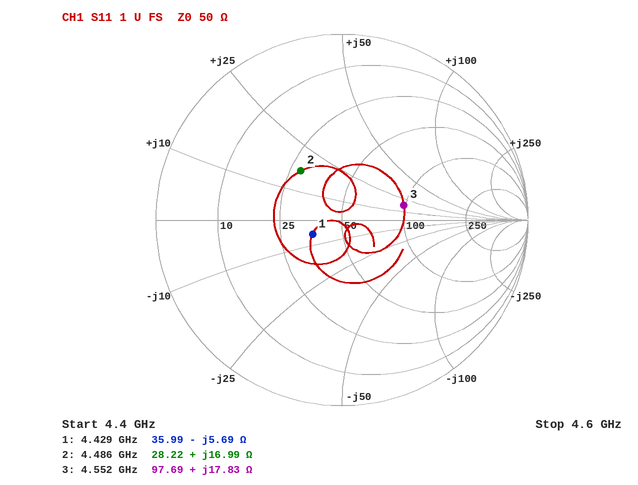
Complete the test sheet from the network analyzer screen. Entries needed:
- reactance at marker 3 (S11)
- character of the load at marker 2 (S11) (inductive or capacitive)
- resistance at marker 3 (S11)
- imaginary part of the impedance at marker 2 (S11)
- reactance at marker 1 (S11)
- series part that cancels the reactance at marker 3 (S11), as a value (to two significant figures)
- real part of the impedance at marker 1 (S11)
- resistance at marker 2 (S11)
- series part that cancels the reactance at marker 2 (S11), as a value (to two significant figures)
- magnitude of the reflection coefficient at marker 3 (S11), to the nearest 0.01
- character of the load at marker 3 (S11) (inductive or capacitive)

+17.83 Ω
inductive
97.69 Ω
+16.99 Ω
-5.69 Ω
2.0 pF
35.99 Ω
28.22 Ω
2.1 pF
0.34
inductive
